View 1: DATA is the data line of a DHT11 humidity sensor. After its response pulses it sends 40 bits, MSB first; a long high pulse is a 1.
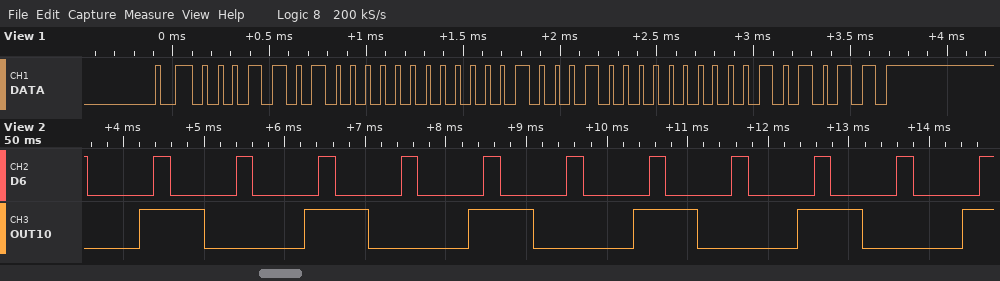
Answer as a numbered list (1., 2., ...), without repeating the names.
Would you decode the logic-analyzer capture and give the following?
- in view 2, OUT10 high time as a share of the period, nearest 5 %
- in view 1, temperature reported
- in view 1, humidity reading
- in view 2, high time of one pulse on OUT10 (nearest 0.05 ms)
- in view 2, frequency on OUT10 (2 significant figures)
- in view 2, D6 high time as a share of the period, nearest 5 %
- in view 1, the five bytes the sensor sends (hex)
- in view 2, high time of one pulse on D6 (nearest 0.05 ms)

1. 40 %
2. 17.0 °C
3. 26 %
4. 0.80 ms
5. 490 Hz
6. 20 %
7. 1A 00 11 00 2B
8. 0.20 ms
